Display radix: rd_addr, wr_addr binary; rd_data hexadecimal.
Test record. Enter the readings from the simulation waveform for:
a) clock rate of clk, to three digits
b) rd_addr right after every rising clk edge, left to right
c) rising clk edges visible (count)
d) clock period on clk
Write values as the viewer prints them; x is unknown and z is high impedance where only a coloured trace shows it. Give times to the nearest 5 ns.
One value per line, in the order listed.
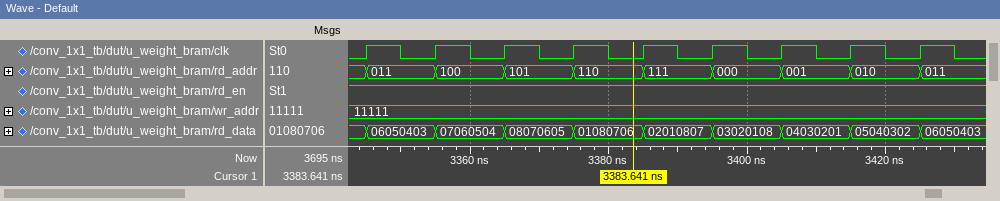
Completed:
100 MHz
011, 100, 101, 110, 111, 000, 001, 010, 011
9
10 ns
